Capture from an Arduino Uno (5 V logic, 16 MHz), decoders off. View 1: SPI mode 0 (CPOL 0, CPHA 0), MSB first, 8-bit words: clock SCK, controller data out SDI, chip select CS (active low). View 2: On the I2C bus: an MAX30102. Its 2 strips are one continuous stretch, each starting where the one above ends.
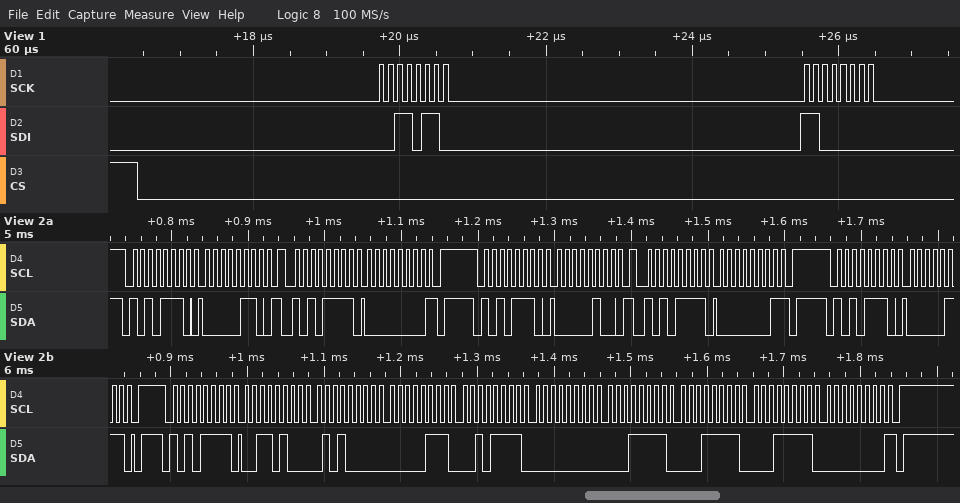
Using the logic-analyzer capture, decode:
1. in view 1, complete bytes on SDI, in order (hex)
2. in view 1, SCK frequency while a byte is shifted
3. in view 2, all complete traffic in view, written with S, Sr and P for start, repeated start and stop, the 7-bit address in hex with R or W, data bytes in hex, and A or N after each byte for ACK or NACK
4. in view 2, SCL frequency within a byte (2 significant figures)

36 C0
8 MHz
S 57W A 06 A Sr 57R A 00 N P S 57W A 04 A Sr 57R A 01 N P S 57W A 07 A P S 57R A 34 A 50 A 07 A 2F A 00 A 1F A 1F A 1F A 00 N P
100 kHz
